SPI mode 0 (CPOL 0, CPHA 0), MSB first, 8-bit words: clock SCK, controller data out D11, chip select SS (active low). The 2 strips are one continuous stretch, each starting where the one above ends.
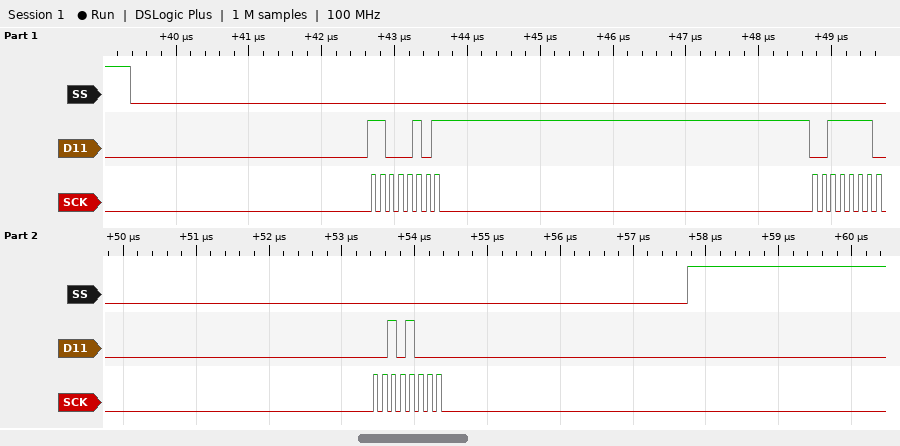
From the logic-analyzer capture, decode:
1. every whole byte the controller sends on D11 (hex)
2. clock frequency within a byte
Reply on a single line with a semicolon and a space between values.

0xC5 0x3E 0x28; 8 MHz
